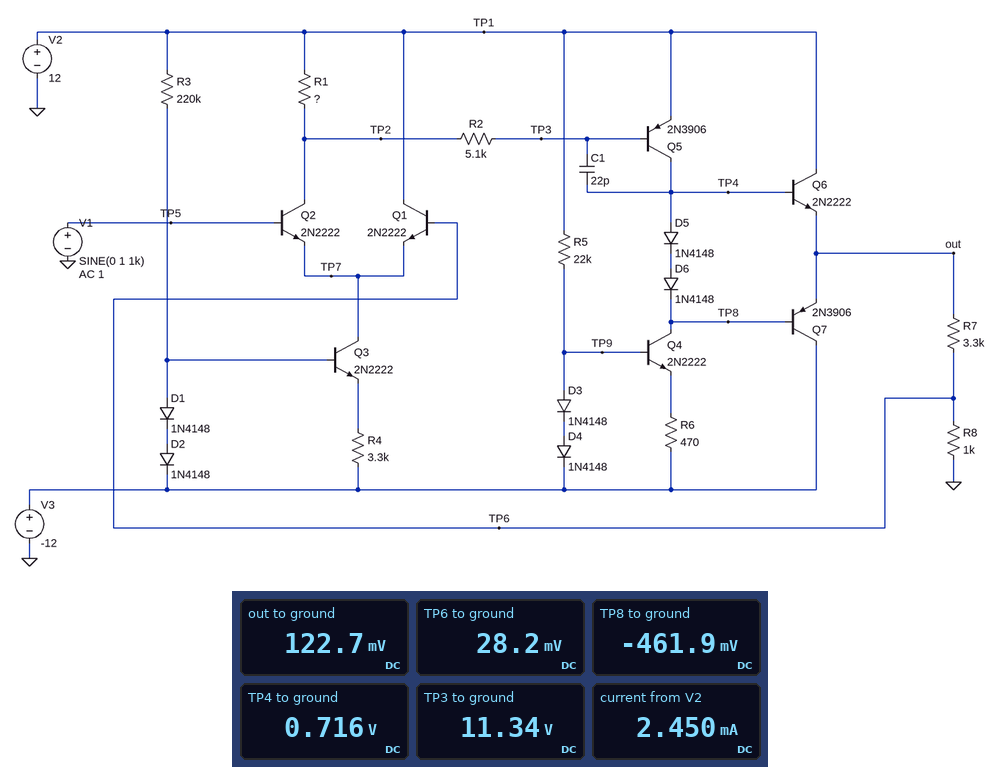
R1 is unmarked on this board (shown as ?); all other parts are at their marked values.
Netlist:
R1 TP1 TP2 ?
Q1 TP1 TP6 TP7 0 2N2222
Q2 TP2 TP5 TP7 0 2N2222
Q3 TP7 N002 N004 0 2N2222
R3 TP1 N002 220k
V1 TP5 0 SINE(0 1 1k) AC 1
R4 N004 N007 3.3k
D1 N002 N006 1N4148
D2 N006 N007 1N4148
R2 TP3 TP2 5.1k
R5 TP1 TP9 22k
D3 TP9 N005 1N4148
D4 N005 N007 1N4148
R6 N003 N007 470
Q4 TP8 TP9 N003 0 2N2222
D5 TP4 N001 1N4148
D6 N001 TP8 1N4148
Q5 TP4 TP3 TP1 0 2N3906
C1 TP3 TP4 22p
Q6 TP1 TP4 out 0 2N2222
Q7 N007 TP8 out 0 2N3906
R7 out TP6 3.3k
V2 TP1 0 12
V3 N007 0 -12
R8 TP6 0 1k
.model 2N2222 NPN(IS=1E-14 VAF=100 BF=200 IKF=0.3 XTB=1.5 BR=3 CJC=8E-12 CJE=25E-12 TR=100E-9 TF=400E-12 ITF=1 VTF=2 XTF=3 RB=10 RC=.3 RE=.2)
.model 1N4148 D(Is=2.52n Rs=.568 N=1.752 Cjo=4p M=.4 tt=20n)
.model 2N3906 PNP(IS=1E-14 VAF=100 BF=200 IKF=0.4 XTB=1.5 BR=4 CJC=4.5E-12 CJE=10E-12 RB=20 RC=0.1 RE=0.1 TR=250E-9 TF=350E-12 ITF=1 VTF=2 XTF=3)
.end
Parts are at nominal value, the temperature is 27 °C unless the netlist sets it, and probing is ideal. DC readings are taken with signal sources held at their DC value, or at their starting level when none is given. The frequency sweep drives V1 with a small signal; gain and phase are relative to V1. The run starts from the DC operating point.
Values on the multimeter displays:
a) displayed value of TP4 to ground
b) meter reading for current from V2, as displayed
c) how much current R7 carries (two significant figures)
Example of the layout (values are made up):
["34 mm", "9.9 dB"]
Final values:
["0.716 V", "2.450 mA", "29 µA"]
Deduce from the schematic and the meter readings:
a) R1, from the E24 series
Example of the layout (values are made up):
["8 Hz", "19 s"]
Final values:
["30 kΩ"]
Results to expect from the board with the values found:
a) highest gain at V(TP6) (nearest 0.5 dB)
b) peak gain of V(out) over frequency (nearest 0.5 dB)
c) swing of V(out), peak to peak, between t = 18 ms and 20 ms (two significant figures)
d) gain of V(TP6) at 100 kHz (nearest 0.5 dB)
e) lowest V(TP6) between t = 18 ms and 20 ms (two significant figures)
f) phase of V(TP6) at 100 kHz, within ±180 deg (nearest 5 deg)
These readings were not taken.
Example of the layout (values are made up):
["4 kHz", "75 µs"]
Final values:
["0 dB", "12.5 dB", "8.6 V", "0 dB", "-970 mV", "-5 deg"]
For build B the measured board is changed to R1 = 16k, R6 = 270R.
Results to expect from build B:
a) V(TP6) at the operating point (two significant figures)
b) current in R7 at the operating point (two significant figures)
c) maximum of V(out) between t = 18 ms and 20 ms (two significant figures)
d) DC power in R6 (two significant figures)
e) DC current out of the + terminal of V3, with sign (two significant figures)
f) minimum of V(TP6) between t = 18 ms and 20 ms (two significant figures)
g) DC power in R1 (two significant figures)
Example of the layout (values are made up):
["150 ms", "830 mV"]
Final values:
["2.0 mV", "2.3 µA", "4.3 V", "940 µW", "-3.3 mA", "-1.0 V", "32 µW"]
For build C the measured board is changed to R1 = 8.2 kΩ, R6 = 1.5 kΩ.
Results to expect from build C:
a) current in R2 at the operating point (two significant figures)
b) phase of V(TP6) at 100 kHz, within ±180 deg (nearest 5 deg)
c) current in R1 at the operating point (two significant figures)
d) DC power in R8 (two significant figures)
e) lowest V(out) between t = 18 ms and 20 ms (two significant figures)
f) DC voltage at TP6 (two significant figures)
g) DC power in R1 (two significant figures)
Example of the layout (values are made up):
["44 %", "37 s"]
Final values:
["1.6 µA", "-10 deg", "77 µA", "580 nW", "-4.4 V", "-24 mV", "49 µW"]
